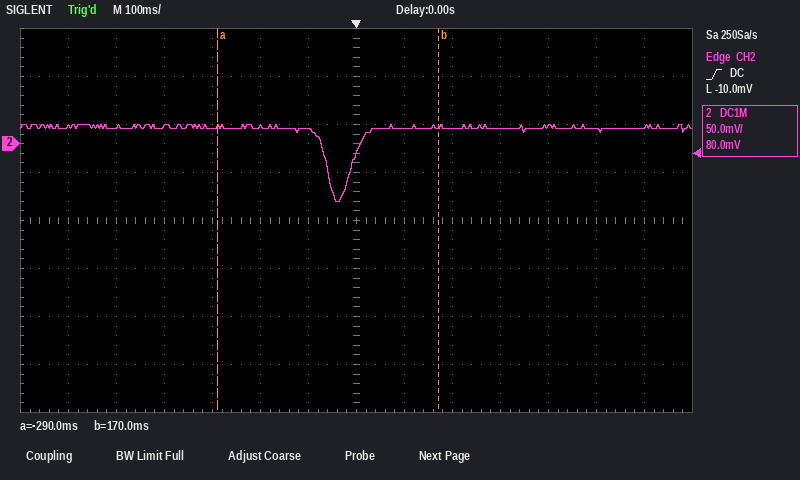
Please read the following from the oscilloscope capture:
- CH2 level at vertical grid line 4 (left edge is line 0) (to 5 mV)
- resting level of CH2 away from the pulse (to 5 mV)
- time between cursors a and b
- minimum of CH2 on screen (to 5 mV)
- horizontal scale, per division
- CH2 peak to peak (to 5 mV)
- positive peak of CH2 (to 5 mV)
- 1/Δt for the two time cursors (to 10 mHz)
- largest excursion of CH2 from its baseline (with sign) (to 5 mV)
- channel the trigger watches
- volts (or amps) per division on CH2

15 mV
15 mV
460 ms
-60 mV
100 ms
80 mV
20 mV
2.17 Hz
-75 mV
CH2
50 mV
